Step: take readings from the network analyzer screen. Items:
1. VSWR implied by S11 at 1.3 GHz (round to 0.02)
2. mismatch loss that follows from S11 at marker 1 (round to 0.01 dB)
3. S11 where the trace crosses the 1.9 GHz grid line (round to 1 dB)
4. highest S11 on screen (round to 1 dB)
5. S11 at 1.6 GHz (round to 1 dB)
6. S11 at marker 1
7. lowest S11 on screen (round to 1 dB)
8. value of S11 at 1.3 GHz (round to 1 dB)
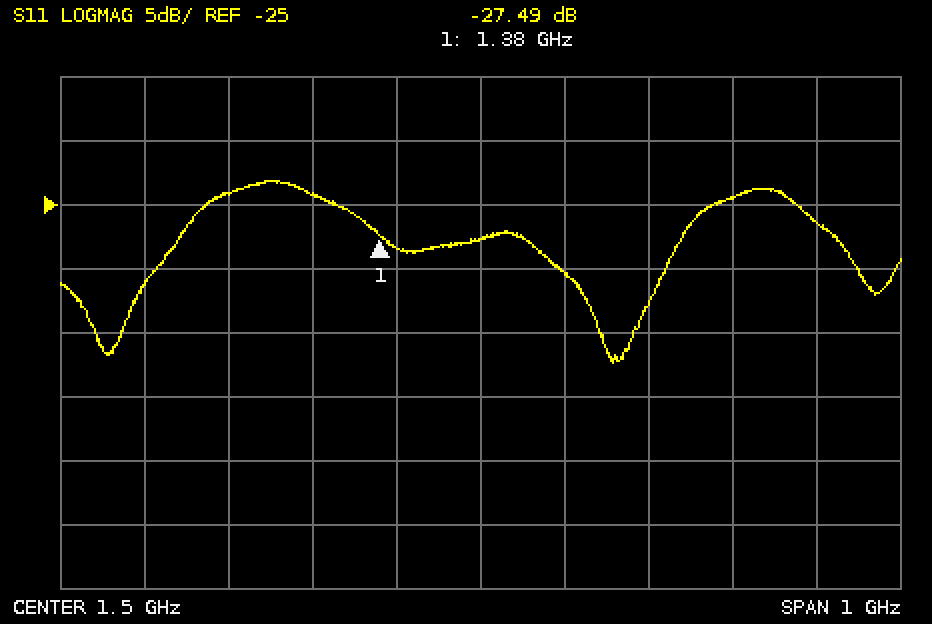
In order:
1.14
0.01 dB
-26 dB
-23 dB
-30 dB
-27.49 dB
-37 dB
-24 dB
